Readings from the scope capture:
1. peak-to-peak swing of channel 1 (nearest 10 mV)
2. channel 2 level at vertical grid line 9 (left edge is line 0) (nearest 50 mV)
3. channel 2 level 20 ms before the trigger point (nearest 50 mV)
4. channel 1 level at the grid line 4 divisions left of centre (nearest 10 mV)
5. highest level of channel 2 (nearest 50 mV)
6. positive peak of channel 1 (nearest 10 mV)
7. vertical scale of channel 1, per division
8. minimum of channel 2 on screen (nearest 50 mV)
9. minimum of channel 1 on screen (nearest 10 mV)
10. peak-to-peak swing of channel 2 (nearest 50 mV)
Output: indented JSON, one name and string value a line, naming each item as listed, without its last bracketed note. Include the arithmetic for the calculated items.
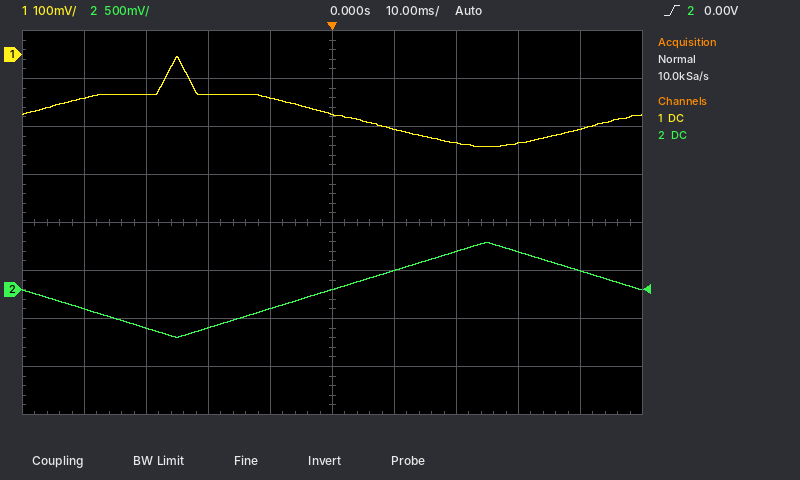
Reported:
{
  "peak-to-peak swing of channel 1": "0 mV − (-190 mV) = 190 mV",
  "channel 2 level at vertical grid line 9 (left edge is line 0)": "200 mV",
  "channel 2 level 20 ms before the trigger point": "-400 mV",
  "channel 1 level at the grid line 4 divisions left of centre": "-90 mV",
  "highest level of channel 2": "500 mV",
  "positive peak of channel 1": "0 mV",
  "vertical scale of channel 1, per division": "100 mV",
  "minimum of channel 2 on screen": "-500 mV",
  "minimum of channel 1 on screen": "-190 mV",
  "peak-to-peak swing of channel 2": "500 mV − (-500 mV) = 1.00 V"
}
